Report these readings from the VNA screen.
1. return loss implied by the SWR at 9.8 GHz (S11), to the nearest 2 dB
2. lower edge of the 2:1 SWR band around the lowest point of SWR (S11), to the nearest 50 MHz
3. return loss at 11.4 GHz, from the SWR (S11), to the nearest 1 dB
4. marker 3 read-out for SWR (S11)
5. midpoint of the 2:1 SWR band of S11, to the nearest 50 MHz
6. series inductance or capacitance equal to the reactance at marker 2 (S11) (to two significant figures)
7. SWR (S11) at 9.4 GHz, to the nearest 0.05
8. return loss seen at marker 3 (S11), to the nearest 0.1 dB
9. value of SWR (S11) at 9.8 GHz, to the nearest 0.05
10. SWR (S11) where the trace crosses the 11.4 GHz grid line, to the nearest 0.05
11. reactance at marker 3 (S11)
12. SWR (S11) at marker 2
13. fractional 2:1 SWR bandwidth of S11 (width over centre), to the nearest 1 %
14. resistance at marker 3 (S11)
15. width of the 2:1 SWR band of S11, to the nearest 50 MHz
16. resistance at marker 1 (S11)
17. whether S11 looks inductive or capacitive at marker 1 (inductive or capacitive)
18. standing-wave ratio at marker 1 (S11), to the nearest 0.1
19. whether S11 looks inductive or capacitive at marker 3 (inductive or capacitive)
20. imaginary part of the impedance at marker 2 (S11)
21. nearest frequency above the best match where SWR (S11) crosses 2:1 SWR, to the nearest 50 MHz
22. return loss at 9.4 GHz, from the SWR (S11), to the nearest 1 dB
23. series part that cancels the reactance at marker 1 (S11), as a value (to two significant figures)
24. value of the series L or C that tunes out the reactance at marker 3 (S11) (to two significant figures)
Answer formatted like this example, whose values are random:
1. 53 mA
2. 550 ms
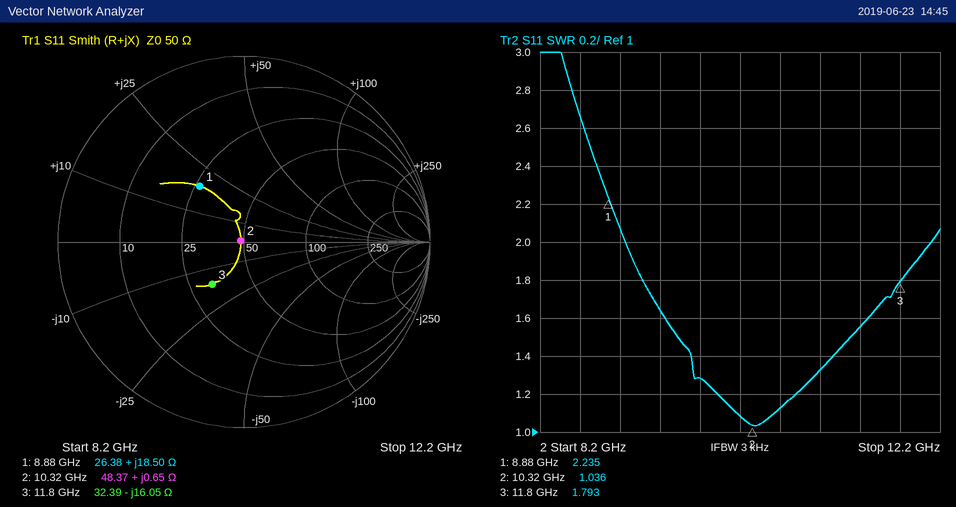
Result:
1. 18 dB
2. 9.05 GHz
3. 13 dB
4. 1.793
5. 10.60 GHz
6. 10 pH
7. 1.65
8. 10.9 dB
9. 1.30
10. 1.55
11. -16.05 Ω
12. 1.036
13. 29 %
14. 32.39 Ω
15. 3.05 GHz
16. 26.38 Ω
17. inductive
18. 2.2
19. capacitive
20. +0.65 Ω
21. 12.10 GHz
22. 12 dB
23. 970 fF
24. 220 pH
